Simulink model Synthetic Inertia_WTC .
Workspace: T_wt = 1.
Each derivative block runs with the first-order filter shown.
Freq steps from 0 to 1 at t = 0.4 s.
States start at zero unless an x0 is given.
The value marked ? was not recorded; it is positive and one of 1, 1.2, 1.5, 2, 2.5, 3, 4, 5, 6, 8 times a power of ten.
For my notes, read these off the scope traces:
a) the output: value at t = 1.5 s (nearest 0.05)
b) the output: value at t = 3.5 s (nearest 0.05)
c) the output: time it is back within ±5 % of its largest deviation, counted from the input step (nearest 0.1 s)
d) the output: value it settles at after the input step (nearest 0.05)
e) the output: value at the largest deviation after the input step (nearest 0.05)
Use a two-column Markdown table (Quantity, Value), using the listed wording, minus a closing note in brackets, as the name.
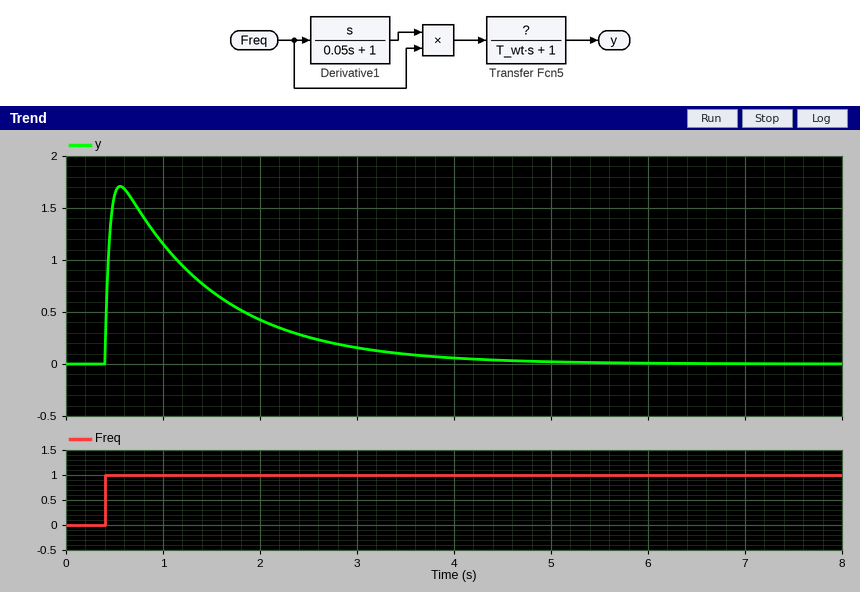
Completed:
| Quantity | Value |
|---|---|
| the output: value at t = 1.5 s | 0.70 |
| the output: value at t = 3.5 s | 0.10 |
| the output: time it is back within ±5 % of its largest deviation, counted from the input step | 3.2 s |
| the output: value it settles at after the input step | 0.00 |
| the output: value at the largest deviation after the input step | 1.70 |
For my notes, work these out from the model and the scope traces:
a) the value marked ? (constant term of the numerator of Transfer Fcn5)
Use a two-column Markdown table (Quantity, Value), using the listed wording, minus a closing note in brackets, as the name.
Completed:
| Quantity | Value |
|---|---|
| the value marked ? | 2 |
